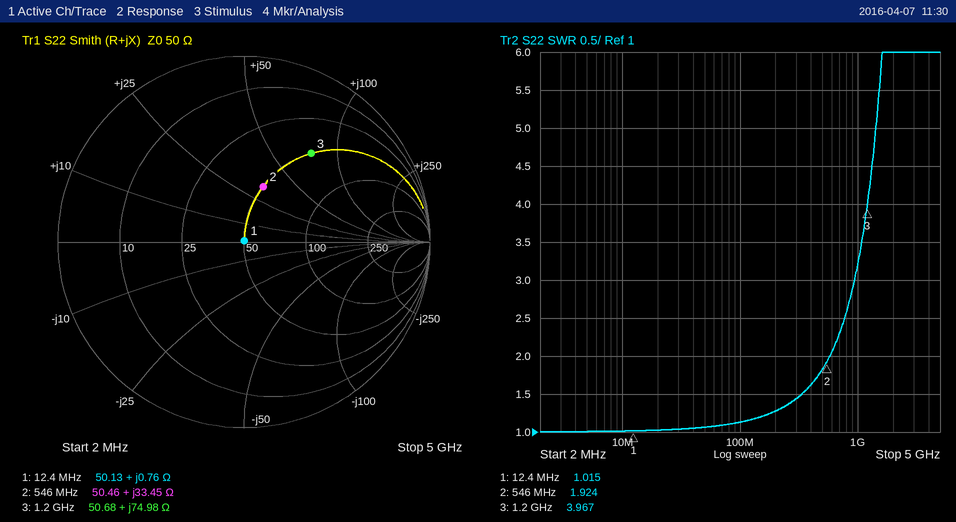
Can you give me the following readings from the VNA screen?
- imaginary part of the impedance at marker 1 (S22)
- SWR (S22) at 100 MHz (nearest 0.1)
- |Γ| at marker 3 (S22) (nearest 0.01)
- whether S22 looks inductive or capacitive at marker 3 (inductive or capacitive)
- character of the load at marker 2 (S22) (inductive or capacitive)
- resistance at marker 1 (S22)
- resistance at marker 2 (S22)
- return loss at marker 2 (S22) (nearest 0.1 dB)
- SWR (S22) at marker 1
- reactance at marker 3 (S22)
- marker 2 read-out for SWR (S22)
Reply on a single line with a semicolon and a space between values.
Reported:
+0.76 Ω; 1.1; 0.60; inductive; inductive; 50.13 Ω; 50.46 Ω; 10.0 dB; 1.015; +74.98 Ω; 1.924
